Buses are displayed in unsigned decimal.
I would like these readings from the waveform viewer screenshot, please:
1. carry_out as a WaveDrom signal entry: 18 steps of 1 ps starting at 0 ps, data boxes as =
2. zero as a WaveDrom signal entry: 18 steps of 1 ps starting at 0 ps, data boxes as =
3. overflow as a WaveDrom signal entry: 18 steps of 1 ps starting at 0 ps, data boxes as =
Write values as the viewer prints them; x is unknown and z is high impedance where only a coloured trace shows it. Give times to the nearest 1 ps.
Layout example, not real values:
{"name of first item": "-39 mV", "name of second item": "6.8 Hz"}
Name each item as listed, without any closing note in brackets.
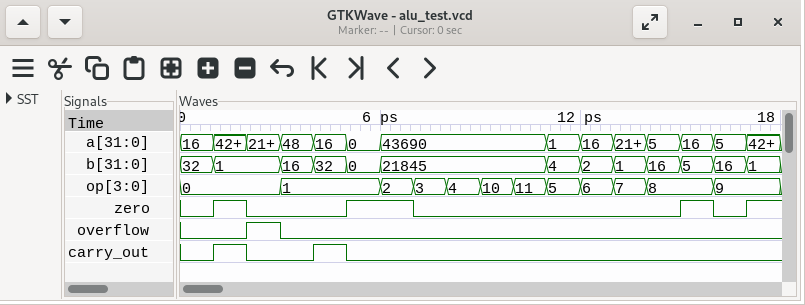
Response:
{"carry_out as a WaveDrom signal entry: 18 steps of 1 ps starting at 0 ps, data boxes as =": "{name: 'carry_out', wave: '010.10............'}", "zero as a WaveDrom signal entry: 18 steps of 1 ps starting at 0 ps, data boxes as =": "{name: 'zero', wave: '010..1.0.......101'}", "overflow as a WaveDrom signal entry: 18 steps of 1 ps starting at 0 ps, data boxes as =": "{name: 'overflow', wave: '0.10..............'}"}
